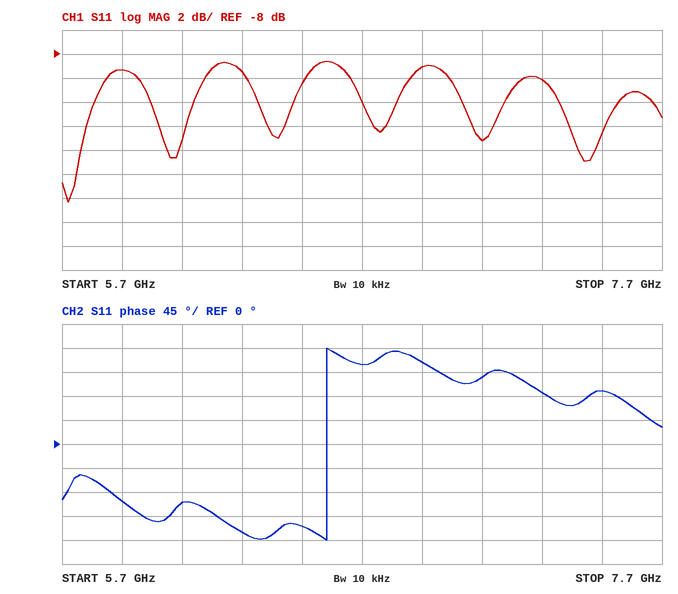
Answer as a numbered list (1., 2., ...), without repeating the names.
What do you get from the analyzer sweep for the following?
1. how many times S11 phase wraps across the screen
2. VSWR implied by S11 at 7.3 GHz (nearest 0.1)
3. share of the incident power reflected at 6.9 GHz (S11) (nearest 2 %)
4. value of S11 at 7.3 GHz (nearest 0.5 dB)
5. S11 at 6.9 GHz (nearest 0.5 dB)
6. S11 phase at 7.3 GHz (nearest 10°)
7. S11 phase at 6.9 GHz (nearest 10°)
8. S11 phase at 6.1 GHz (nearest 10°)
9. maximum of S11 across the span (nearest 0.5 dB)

1. 1
2. 1.9
3. 12 %
4. -10.0 dB
5. -9.0 dB
6. 100°
7. 150°
8. -110°
9. -8.5 dB
